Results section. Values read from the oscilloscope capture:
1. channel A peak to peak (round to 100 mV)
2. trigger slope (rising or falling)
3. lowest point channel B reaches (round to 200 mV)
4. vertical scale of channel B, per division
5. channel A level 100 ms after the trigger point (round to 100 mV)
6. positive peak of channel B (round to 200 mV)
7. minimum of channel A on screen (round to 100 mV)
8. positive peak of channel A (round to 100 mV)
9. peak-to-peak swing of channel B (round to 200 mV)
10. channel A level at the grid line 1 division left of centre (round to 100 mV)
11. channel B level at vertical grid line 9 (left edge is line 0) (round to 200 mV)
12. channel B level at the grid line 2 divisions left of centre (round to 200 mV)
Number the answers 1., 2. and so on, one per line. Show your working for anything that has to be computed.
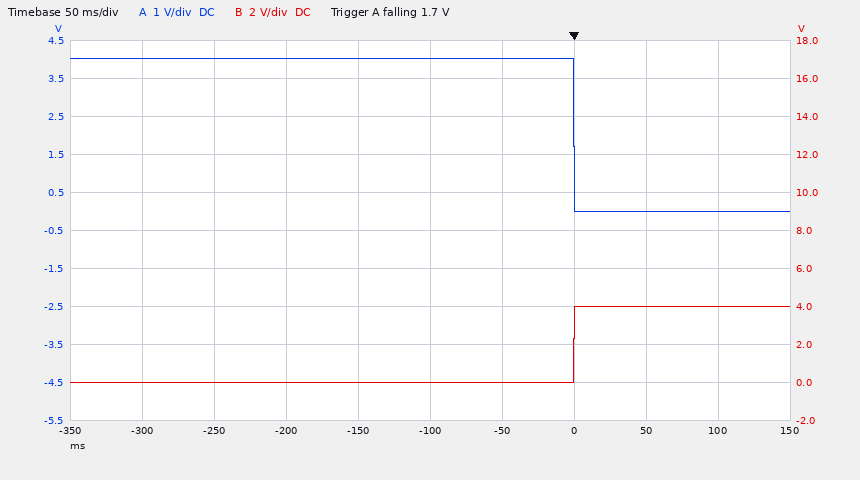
1. 4.0 V − (0.0 V) = 4.0 V
2. falling
3. 0.0 V
4. 2 V
5. 0.0 V
6. 4.0 V
7. 0.0 V
8. 4.0 V
9. 4.0 V − (0.0 V) = 4.0 V
10. 4.0 V
11. 4.0 V
12. 0.0 V
